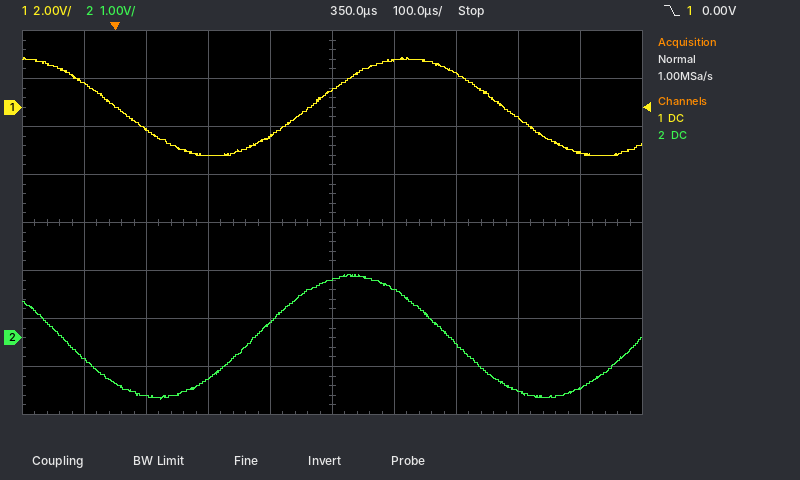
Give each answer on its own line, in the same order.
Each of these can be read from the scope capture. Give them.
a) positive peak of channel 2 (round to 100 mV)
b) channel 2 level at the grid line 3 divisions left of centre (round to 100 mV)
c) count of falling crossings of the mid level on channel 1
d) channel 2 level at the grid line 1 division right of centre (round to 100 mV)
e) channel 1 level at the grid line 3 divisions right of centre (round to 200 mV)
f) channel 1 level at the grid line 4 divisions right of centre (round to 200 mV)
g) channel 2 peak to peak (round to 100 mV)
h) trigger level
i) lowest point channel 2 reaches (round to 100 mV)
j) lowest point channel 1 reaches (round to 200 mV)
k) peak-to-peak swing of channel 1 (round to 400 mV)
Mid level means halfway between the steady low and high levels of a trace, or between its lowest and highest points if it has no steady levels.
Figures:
1.3 V
-1.2 V
2
1.0 V
-400 mV
-1.8 V
2.6 V
0.00 V
-1.3 V
-2.0 V
4.0 V
